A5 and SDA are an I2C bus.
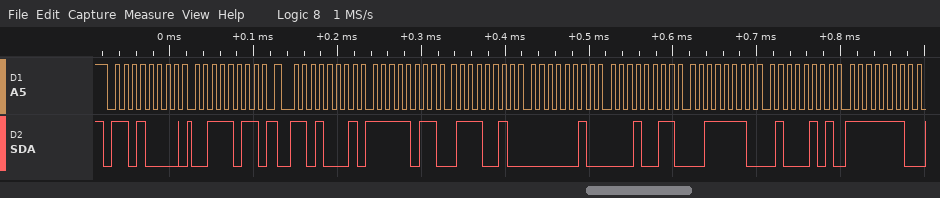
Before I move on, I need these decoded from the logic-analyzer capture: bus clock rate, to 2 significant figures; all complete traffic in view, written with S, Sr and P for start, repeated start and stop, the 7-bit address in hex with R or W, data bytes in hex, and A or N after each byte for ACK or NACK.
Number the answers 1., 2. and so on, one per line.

1. 100 kHz
2. S 68W A 3B A Sr 68R A FB A 72 A 02 A 13 A 3E A 45 A FE A
